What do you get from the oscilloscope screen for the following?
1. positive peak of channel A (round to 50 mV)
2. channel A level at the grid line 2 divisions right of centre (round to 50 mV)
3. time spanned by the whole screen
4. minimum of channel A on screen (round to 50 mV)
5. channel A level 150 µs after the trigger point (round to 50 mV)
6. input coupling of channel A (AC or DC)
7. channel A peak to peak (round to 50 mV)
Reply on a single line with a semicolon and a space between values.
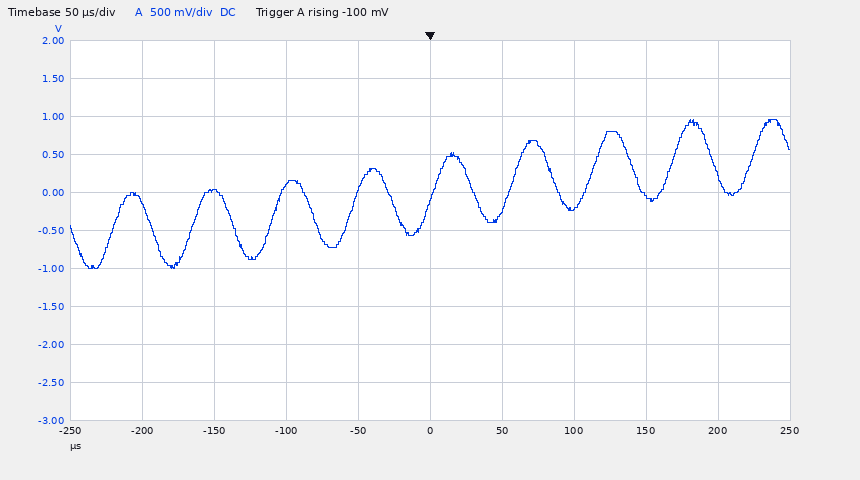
950 mV; -200 mV; 500 µs; -1.00 V; -50 mV; DC; 1.95 V
